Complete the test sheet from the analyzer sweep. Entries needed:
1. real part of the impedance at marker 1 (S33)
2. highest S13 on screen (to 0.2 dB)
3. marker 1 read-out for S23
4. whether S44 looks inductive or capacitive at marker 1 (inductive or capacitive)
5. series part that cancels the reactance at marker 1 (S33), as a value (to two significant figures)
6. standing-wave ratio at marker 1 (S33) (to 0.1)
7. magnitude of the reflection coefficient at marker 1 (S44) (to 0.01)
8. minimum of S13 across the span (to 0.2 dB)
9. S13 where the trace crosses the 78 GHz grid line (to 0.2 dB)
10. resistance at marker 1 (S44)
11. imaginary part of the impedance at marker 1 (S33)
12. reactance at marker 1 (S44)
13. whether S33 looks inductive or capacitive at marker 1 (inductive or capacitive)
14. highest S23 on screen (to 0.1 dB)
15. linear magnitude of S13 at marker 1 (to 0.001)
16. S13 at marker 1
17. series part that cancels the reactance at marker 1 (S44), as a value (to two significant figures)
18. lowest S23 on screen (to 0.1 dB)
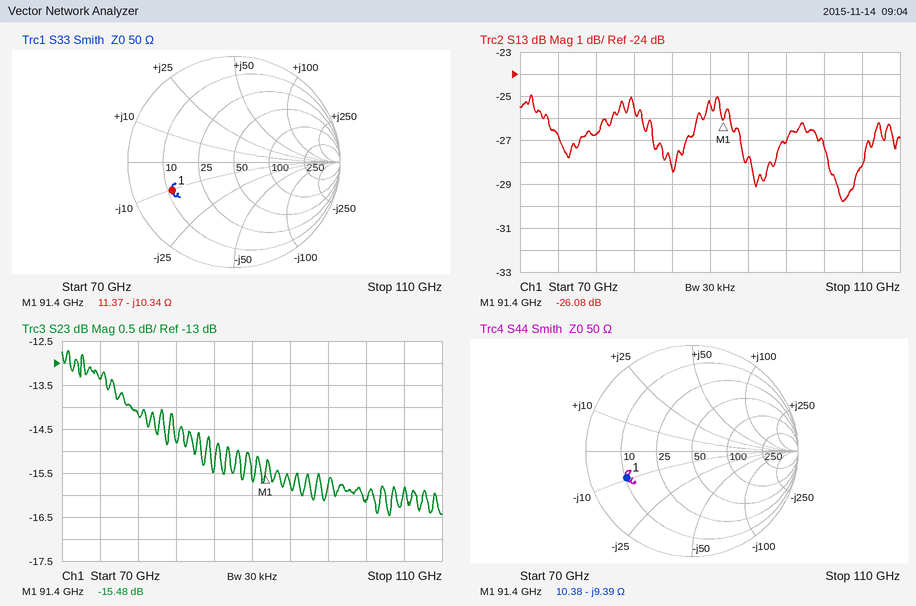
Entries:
11.37 Ω
-25.0 dB
-15.48 dB
capacitive
18 pH
4.6
0.67
-29.8 dB
-26.8 dB
10.38 Ω
-10.34 Ω
-9.39 Ω
capacitive
-12.7 dB
0.050
-26.08 dB
16 pH
-16.5 dB
